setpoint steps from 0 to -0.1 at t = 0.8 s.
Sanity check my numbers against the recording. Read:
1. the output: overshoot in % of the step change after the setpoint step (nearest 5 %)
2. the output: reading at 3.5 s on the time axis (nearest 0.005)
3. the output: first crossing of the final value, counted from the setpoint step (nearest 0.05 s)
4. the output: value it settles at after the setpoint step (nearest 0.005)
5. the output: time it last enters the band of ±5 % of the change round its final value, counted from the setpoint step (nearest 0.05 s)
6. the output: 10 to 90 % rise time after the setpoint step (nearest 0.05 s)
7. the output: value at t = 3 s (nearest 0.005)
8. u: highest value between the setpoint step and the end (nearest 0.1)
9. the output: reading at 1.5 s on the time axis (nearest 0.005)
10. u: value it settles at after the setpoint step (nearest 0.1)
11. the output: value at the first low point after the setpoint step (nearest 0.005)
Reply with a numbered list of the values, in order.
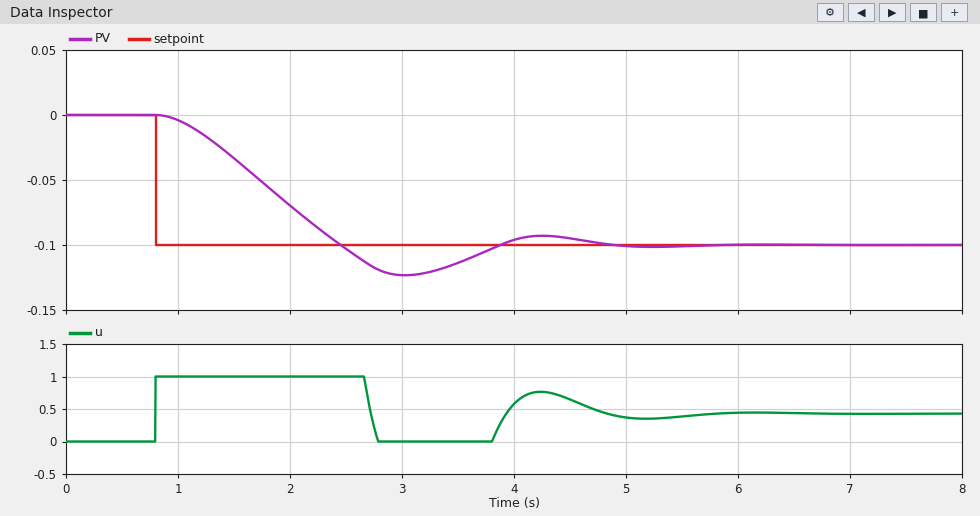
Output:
1. 25 %
2. -0.115
3. 1.65 s
4. -0.100
5. 3.70 s
6. 1.15 s
7. -0.125
8. 1.0
9. -0.035
10. 0.4
11. -0.125
